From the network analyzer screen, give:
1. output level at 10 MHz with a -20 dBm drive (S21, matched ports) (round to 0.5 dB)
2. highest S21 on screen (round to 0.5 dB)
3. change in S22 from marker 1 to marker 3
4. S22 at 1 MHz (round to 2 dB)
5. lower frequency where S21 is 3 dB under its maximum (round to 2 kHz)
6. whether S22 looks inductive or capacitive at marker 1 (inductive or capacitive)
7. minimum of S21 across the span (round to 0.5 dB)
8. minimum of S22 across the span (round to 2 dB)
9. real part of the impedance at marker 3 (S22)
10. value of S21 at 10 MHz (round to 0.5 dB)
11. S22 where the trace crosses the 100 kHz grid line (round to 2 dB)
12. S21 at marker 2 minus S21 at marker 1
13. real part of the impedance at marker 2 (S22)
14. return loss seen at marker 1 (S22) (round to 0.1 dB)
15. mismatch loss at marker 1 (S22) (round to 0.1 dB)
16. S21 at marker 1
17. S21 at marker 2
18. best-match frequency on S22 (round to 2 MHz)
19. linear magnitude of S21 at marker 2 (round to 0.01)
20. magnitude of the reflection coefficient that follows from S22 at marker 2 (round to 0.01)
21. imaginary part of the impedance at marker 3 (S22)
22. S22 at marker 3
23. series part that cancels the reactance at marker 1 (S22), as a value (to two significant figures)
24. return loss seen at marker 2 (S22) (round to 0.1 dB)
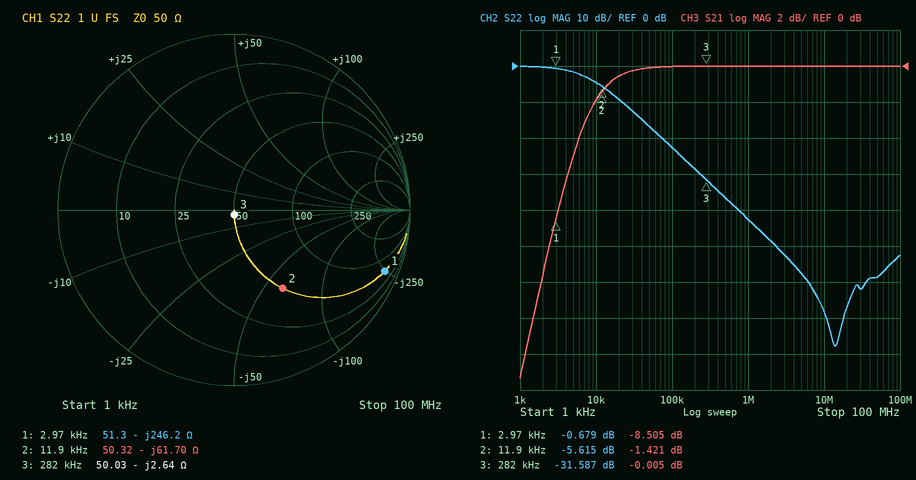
-20.0 dBm
0.0 dB
-30.908 dB
-42 dB
8 kHz
capacitive
-17.5 dB
-78 dB
50.03 Ω
0.0 dB
-22 dB
7.084 dB
50.32 Ω
0.7 dB
8.4 dB
-8.505 dB
-1.421 dB
14 MHz
0.85
0.52
-2.64 Ω
-31.587 dB
13 mH
5.6 dB
